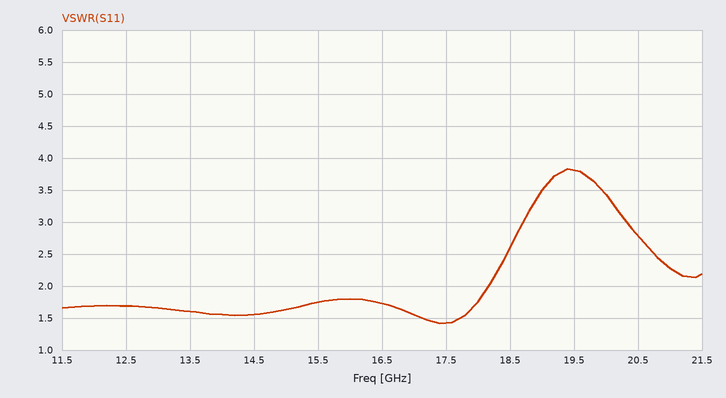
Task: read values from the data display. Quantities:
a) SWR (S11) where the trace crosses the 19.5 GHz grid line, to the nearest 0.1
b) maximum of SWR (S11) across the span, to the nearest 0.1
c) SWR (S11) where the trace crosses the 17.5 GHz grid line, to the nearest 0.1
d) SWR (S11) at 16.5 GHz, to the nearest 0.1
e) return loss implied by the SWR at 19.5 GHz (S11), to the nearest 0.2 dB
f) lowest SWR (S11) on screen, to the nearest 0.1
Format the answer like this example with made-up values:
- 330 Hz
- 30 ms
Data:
- 3.8
- 3.8
- 1.4
- 1.7
- 4.6 dB
- 1.4
